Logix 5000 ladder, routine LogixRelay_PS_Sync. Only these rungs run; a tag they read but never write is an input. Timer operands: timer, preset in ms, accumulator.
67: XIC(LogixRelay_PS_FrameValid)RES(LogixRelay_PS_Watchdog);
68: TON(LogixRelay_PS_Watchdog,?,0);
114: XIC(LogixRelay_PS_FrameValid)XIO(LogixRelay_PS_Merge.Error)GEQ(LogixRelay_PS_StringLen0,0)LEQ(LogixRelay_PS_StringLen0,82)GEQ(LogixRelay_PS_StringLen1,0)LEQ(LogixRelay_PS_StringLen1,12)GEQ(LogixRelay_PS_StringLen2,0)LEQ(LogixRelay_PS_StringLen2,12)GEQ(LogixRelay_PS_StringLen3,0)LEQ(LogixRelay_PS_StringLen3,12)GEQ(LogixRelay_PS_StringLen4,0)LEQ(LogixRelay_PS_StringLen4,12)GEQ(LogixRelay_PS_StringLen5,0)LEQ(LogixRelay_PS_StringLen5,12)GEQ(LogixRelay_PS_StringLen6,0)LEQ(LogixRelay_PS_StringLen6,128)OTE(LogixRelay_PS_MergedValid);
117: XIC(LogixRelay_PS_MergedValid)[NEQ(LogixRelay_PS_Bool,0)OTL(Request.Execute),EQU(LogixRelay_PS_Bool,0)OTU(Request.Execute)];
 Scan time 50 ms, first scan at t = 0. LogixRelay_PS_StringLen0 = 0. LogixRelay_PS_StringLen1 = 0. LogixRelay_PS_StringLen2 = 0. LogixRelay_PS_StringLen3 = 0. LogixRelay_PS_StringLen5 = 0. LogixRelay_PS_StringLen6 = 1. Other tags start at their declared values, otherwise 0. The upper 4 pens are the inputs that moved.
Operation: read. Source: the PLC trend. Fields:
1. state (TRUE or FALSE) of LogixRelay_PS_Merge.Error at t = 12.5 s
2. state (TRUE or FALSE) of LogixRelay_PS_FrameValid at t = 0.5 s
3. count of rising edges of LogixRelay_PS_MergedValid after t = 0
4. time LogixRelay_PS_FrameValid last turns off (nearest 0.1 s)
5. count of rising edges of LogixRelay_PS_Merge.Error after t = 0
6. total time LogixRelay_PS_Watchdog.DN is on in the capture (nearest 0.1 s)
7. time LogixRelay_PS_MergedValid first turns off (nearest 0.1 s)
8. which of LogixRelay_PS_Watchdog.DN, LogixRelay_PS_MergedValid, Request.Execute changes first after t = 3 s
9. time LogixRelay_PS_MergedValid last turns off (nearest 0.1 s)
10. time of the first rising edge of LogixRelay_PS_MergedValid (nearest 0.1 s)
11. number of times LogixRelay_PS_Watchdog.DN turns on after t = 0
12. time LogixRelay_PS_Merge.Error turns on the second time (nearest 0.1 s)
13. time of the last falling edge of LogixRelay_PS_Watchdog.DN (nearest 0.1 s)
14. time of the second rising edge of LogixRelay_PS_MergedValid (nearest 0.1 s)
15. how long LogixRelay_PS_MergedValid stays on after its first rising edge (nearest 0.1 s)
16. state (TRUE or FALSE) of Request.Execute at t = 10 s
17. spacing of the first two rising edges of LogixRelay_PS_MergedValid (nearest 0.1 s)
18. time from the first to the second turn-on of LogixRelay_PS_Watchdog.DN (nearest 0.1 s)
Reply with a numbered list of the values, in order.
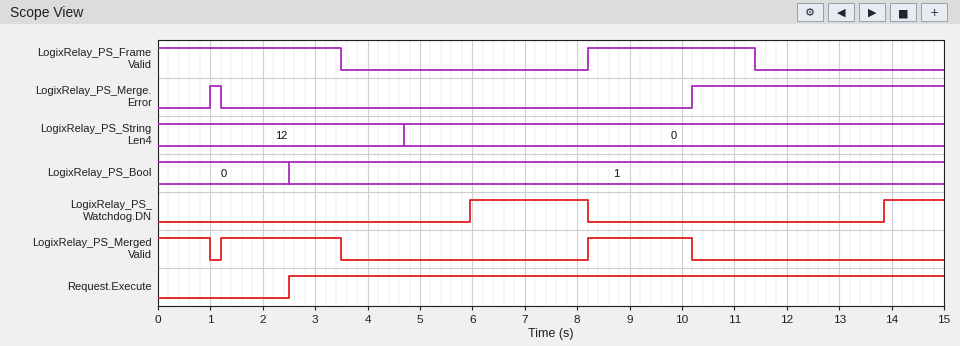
1. TRUE
2. TRUE
3. 2
4. 11.4 s
5. 2
6. 3.4 s
7. 1.0 s
8. LogixRelay_PS_MergedValid
9. 10.2 s
10. 1.2 s
11. 2
12. 10.2 s
13. 8.2 s
14. 8.2 s
15. 2.3 s
16. TRUE
17. 7.0 s
18. 7.9 s
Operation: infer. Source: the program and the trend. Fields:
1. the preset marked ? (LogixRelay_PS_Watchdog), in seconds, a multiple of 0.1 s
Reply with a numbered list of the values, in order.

1. 2.5 s
